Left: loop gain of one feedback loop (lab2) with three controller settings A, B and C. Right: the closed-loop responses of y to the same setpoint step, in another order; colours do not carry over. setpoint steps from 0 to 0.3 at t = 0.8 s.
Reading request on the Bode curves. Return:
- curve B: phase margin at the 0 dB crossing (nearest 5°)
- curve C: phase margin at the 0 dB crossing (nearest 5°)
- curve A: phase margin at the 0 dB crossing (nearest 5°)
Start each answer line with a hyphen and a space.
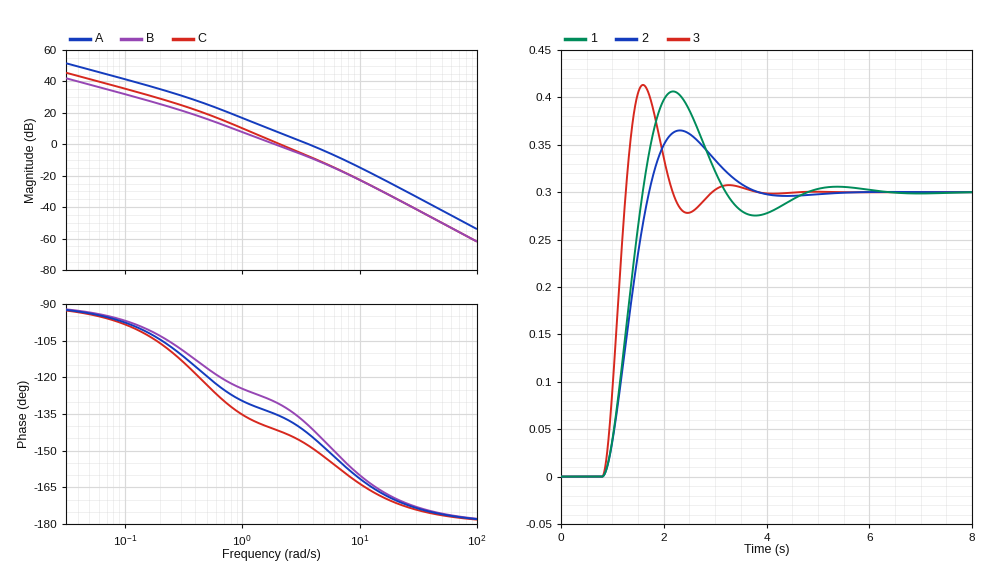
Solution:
- 50°
- 40°
- 35°
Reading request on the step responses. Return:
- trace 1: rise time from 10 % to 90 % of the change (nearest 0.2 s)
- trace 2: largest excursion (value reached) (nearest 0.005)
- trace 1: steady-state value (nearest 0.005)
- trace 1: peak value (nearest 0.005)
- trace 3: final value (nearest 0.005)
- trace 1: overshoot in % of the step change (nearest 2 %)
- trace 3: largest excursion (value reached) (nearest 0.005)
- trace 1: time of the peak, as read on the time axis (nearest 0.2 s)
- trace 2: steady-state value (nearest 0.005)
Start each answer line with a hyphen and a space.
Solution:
- 0.6 s
- 0.365
- 0.300
- 0.405
- 0.300
- 36 %
- 0.415
- 2.2 s
- 0.300
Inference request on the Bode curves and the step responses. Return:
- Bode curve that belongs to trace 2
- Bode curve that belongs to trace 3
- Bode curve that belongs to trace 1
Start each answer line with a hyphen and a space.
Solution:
- B
- A
- C
